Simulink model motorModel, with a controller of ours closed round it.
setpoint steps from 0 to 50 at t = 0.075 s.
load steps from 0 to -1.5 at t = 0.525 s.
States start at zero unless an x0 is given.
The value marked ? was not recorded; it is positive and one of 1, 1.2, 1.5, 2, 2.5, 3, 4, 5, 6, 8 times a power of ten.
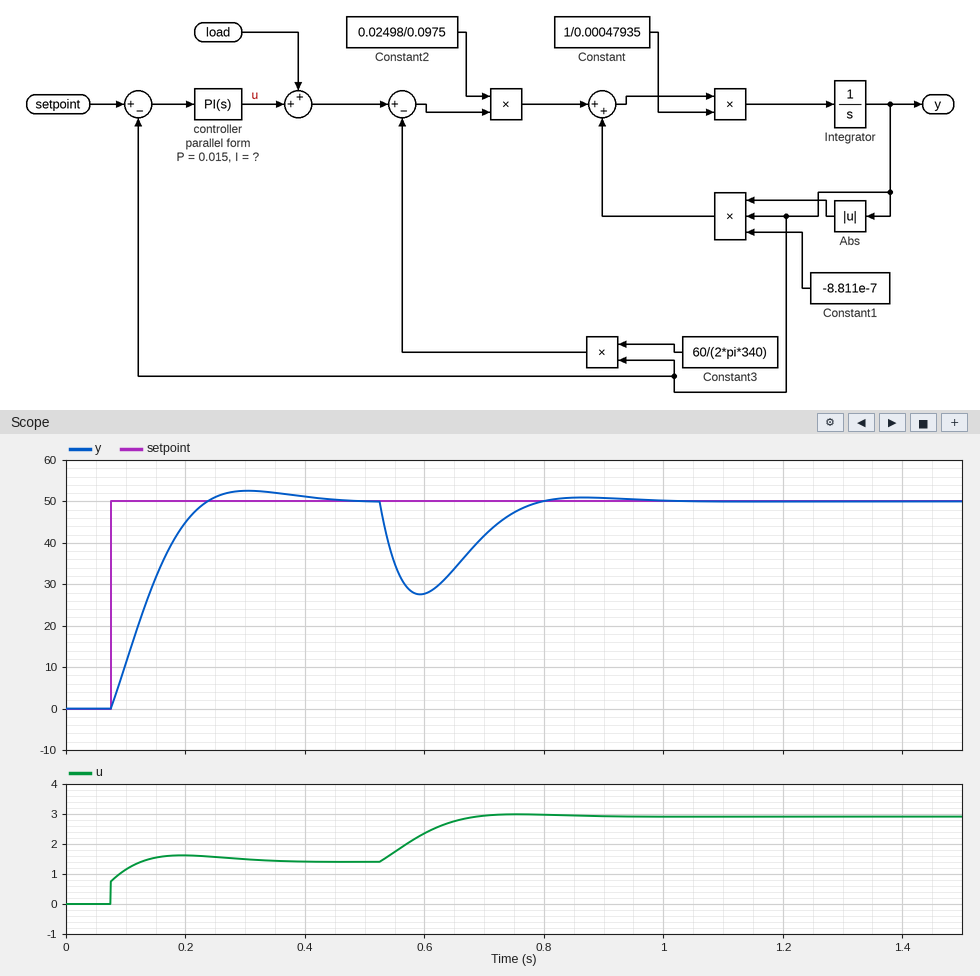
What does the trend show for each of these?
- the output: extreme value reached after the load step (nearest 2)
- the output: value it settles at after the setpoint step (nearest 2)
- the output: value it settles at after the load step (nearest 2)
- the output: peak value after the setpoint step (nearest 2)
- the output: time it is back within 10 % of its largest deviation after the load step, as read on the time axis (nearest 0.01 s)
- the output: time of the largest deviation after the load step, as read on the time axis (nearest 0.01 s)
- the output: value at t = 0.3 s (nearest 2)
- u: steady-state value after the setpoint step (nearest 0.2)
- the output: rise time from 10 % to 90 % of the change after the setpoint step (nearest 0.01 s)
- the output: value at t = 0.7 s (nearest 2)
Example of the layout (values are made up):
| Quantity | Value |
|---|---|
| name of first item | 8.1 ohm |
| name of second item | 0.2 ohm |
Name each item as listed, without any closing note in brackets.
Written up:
| Quantity | Value |
|---|---|
| the output: extreme value reached after the load step | 28 |
| the output: value it settles at after the setpoint step | 50 |
| the output: value it settles at after the load step | 50 |
| the output: peak value after the setpoint step | 52 |
| the output: time it is back within 10 % of its largest deviation after the load step, as read on the time axis | 0.76 s |
| the output: time of the largest deviation after the load step, as read on the time axis | 0.59 s |
| the output: value at t = 0.3 s | 52 |
| u: steady-state value after the setpoint step | 1.4 |
| the output: rise time from 10 % to 90 % of the change after the setpoint step | 0.11 s |
| the output: value at t = 0.7 s | 42 |
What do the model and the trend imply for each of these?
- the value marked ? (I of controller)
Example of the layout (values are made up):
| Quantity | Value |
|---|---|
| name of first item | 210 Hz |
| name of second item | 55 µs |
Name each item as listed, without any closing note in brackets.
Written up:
| Quantity | Value |
|---|---|
| the value marked ? | 0.5 |
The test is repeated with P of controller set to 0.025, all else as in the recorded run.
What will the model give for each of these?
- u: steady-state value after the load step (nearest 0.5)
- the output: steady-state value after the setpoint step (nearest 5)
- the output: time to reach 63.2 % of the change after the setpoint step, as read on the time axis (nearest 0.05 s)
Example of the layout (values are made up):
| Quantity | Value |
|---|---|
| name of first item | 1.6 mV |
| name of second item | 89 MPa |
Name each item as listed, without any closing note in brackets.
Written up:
| Quantity | Value |
|---|---|
| u: steady-state value after the load step | 3.0 |
| the output: steady-state value after the setpoint step | 50 |
| the output: time to reach 63.2 % of the change after the setpoint step, as read on the time axis | 0.15 s |
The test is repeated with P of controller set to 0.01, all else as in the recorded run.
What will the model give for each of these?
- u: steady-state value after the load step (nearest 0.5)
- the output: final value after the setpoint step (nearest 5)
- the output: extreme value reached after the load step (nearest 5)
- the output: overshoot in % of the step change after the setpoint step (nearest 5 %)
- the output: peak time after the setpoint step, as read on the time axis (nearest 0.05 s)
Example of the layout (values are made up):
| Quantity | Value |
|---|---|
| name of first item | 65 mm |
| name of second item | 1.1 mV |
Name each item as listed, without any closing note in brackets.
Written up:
| Quantity | Value |
|---|---|
| u: steady-state value after the load step | 3.0 |
| the output: final value after the setpoint step | 50 |
| the output: extreme value reached after the load step | 25 |
| the output: overshoot in % of the step change after the setpoint step | 10 % |
| the output: peak time after the setpoint step, as read on the time axis | 0.30 s |
